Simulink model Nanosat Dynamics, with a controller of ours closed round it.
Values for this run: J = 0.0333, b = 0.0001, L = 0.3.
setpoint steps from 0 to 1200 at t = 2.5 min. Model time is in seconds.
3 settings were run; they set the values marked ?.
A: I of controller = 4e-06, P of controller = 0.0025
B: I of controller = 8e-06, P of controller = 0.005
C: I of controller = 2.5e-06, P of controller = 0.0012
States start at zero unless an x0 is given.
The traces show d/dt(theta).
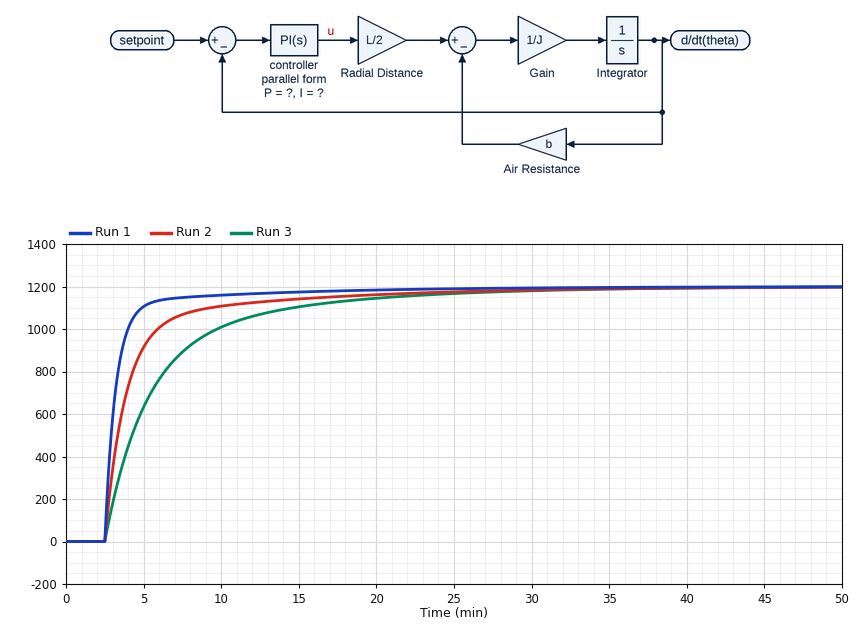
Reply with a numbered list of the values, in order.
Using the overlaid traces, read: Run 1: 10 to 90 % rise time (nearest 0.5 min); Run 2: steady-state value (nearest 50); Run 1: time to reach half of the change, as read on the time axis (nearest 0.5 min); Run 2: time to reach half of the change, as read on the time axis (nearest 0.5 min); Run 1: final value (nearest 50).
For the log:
1. 2.0 min
2. 1200
3. 3.0 min
4. 3.5 min
5. 1200
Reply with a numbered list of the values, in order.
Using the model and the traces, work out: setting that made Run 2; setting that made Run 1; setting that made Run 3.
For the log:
1. A
2. B
3. C
